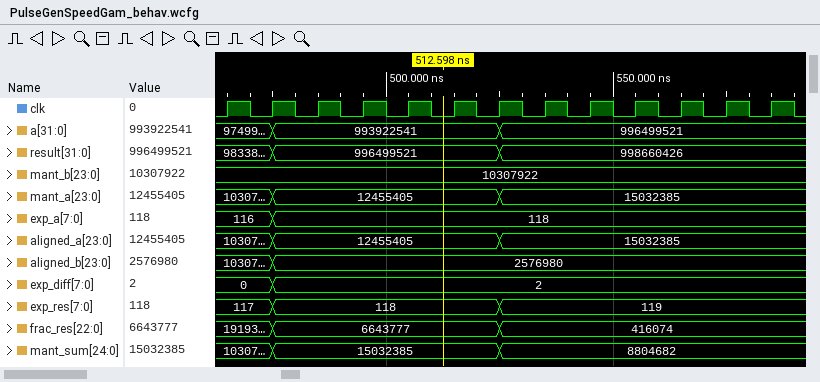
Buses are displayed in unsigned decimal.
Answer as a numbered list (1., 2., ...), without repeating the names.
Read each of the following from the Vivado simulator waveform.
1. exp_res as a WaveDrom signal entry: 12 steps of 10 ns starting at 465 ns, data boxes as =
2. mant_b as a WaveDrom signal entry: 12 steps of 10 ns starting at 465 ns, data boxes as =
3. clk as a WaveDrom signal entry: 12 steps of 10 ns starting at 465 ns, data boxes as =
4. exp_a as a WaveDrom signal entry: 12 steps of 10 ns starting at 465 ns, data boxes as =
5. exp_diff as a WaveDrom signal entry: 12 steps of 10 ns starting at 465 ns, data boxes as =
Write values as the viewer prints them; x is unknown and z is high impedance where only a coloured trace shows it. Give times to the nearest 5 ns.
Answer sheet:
1. {name: 'exp_res', wave: '==....=.....', data: '117 118 119'}
2. {name: 'mant_b', wave: '=...........', data: '10307922'}
3. {name: 'clk', wave: 'p...........'}
4. {name: 'exp_a', wave: '==..........', data: '116 118'}
5. {name: 'exp_diff', wave: '==..........', data: '0 2'}
